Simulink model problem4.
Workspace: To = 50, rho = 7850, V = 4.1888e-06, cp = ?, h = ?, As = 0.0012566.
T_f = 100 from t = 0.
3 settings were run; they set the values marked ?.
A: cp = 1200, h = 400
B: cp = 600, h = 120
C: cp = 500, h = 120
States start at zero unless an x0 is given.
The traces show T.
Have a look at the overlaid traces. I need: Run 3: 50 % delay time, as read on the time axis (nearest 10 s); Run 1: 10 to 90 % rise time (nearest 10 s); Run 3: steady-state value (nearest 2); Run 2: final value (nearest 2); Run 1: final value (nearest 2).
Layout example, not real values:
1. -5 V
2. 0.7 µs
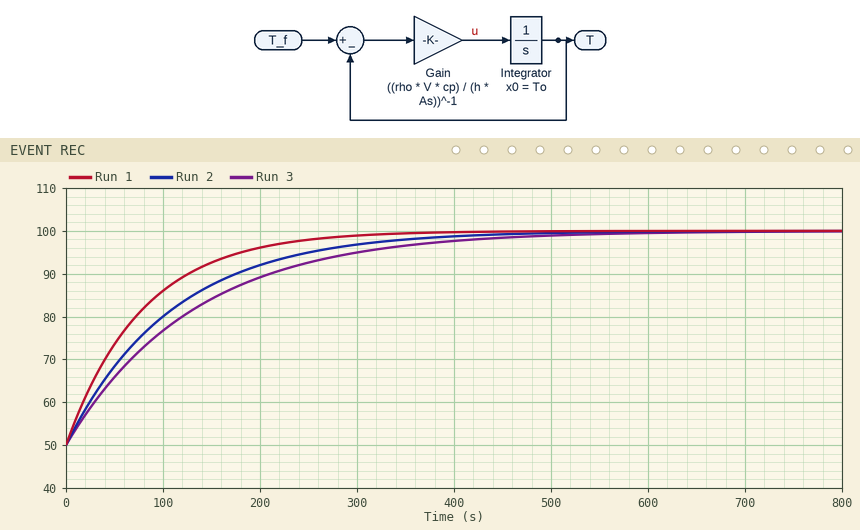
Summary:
1. 90 s
2. 170 s
3. 100
4. 100
5. 100
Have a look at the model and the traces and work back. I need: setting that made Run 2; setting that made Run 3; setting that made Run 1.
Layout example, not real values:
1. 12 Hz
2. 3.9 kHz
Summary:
1. C
2. B
3. A
